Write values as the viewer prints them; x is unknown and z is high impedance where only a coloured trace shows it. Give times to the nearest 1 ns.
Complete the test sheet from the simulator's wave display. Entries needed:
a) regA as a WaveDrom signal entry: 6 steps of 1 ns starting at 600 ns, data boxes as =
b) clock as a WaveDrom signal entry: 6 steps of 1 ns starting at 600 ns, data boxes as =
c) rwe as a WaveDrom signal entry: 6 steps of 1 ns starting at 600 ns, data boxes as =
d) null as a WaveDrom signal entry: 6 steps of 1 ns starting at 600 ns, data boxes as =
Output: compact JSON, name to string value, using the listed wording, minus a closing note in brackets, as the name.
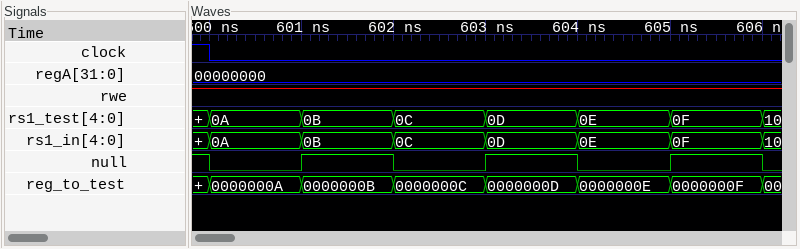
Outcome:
{"regA as a WaveDrom signal entry: 6 steps of 1 ns starting at 600 ns, data boxes as =": "{name: 'regA', wave: '=.....', data: '00000000'}", "clock as a WaveDrom signal entry: 6 steps of 1 ns starting at 600 ns, data boxes as =": "{name: 'clock', wave: '0.....'}", "rwe as a WaveDrom signal entry: 6 steps of 1 ns starting at 600 ns, data boxes as =": "{name: 'rwe', wave: '1.....'}", "null as a WaveDrom signal entry: 6 steps of 1 ns starting at 600 ns, data boxes as =": "{name: 'null', wave: '010101'}"}
